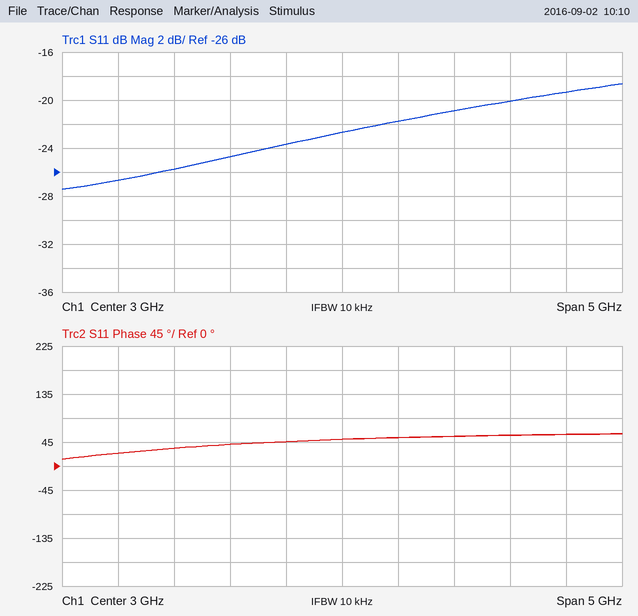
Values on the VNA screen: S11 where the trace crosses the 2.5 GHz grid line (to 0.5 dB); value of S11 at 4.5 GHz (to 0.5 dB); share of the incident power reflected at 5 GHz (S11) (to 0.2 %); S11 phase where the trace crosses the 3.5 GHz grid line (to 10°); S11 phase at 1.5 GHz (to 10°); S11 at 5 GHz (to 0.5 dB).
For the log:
-23.5 dB
-20.0 dB
1.2 %
50°
30°
-19.5 dB
